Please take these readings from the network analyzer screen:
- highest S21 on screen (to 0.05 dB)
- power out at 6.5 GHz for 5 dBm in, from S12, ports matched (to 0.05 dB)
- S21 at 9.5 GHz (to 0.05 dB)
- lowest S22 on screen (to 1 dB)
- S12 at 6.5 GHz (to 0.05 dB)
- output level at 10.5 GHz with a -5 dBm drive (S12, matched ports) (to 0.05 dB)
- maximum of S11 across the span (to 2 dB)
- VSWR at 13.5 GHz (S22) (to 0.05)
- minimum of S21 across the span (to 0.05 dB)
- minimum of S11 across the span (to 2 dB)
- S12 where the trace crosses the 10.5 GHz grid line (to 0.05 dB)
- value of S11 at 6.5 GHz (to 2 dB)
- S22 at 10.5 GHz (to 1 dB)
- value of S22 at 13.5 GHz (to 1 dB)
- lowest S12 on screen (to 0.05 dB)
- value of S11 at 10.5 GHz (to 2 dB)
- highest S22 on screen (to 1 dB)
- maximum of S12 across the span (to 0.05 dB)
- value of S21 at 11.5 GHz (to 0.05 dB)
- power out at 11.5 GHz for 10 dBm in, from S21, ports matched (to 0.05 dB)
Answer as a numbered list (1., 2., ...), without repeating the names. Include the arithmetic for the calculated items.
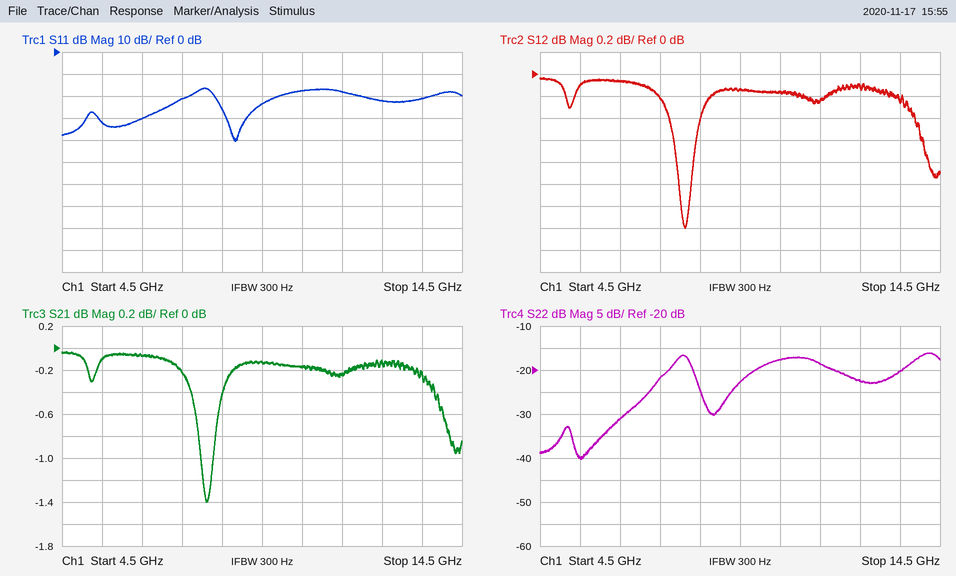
1. -0.05 dB
2. 5 dBm + (-0.05 dB) = 4.95 dBm
3. -0.15 dB
4. -40 dB
5. -0.05 dB
6. -5 dBm + (-0.15 dB) = -5.15 dBm
7. -16 dB
8. |Γ| = 10^(-20/20) = 0.1000; VSWR = (1 + 0.1000)/(1 − 0.1000) ≈ 1.22, so 1.20 to the nearest 0.05
9. -1.40 dB
10. -40 dB
11. -0.15 dB
12. -30 dB
13. -18 dB
14. -20 dB
15. -1.40 dB
16. -18 dB
17. -16 dB
18. -0.05 dB
19. -0.25 dB
20. 10 dBm + (-0.25 dB) = 9.75 dBm
